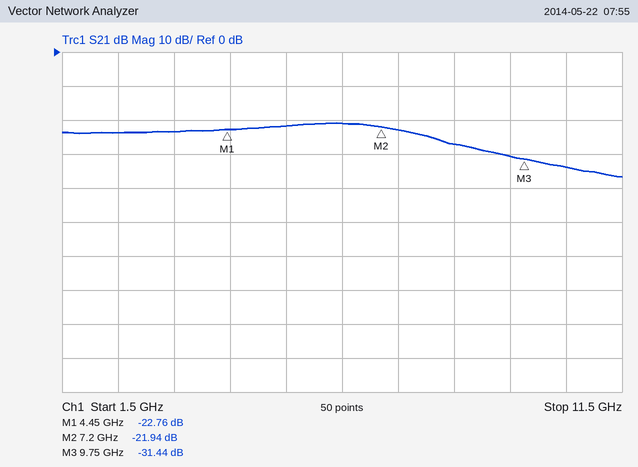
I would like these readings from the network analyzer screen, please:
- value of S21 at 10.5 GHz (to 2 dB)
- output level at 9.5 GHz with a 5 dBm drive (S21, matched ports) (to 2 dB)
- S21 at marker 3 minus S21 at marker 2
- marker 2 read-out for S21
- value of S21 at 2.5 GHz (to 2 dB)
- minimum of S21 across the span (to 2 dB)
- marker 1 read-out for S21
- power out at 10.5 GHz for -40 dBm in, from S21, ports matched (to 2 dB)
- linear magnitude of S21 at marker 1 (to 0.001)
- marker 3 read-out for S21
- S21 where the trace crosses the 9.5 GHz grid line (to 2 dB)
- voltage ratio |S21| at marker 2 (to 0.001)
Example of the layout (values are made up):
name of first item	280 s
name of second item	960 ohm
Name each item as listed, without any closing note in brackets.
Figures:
value of S21 at 10.5 GHz	-34 dB
output level at 9.5 GHz with a 5 dBm drive (S21, matched ports)	-26 dBm
S21 at marker 3 minus S21 at marker 2	-9.50 dB
marker 2 read-out for S21	-21.94 dB
value of S21 at 2.5 GHz	-24 dB
minimum of S21 across the span	-36 dB
marker 1 read-out for S21	-22.76 dB
power out at 10.5 GHz for -40 dBm in, from S21, ports matched	-74 dBm
linear magnitude of S21 at marker 1	0.073
marker 3 read-out for S21	-31.44 dB
S21 where the trace crosses the 9.5 GHz grid line	-30 dB
voltage ratio |S21| at marker 2	0.080
